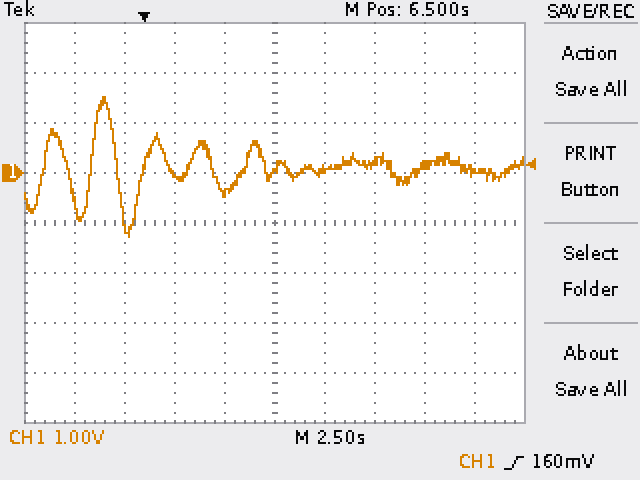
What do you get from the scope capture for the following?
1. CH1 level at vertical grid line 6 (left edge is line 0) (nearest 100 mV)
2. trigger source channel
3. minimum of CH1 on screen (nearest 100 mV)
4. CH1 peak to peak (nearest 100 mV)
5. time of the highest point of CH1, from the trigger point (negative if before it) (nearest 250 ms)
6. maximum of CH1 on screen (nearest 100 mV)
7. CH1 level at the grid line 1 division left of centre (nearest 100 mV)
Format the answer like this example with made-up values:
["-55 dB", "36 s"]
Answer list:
["100 mV", "CH1", "-1.3 V", "2.8 V", "-2.00 s", "1.5 V", "-400 mV"]
